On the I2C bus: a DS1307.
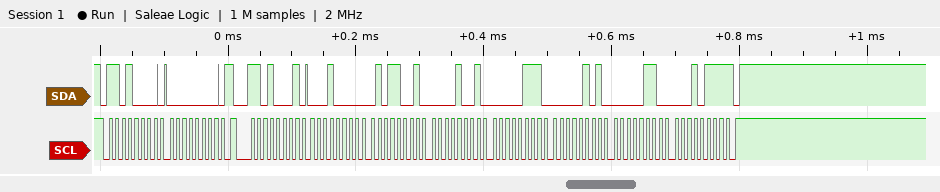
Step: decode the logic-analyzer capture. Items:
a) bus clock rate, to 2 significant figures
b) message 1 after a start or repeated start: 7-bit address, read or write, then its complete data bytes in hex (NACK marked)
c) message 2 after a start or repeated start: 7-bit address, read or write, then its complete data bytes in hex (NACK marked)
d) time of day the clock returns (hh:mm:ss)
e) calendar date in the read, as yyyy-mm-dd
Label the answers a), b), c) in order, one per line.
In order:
a) 100 kHz
b) 0x68 write: 00
c) 0x68 read: 10 59 09 07 05 06 17 NACK
d) 09:59:10
e) 2017-06-05
